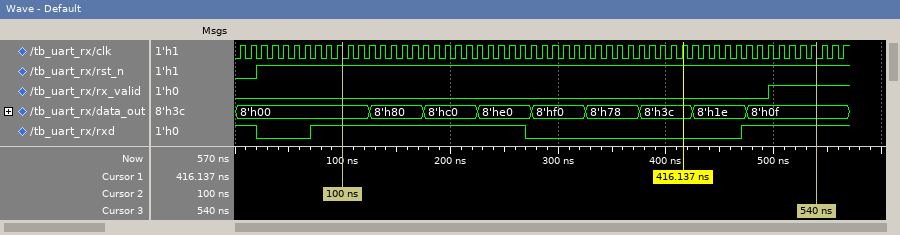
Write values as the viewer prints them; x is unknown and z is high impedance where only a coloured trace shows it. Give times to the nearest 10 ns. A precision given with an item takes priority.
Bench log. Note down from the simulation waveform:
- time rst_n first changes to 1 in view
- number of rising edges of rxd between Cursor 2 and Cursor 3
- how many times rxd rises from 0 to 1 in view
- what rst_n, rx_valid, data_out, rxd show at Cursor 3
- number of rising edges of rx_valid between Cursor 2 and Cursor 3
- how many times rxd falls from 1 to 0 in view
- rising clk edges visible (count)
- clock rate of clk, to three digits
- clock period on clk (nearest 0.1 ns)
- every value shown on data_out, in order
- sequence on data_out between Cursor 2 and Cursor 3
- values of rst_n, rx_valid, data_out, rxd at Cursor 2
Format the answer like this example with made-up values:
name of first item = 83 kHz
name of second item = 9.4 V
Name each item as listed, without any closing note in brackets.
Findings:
time rst_n first changes to 1 in view = 20 ns
number of rising edges of rxd between Cursor 2 and Cursor 3 = 1
how many times rxd rises from 0 to 1 in view = 2
what rst_n, rx_valid, data_out, rxd show at Cursor 3 = rst_n=1, rx_valid=1, data_out=8'h0f, rxd=1
number of rising edges of rx_valid between Cursor 2 and Cursor 3 = 1
how many times rxd falls from 1 to 0 in view = 2
rising clk edges visible = 57
clock rate of clk, to three digits = 100 MHz
clock period on clk = 10 ns
every value shown on data_out, in order = 8'h00, 8'h80, 8'hc0, 8'he0, 8'hf0, 8'h78, 8'h3c, 8'h1e, 8'h0f
sequence on data_out between Cursor 2 and Cursor 3 = 8'h00, 8'h80, 8'hc0, 8'he0, 8'hf0, 8'h78, 8'h3c, 8'h1e, 8'h0f
values of rst_n, rx_valid, data_out, rxd at Cursor 2 = rst_n=1, rx_valid=0, data_out=8'h00, rxd=1
